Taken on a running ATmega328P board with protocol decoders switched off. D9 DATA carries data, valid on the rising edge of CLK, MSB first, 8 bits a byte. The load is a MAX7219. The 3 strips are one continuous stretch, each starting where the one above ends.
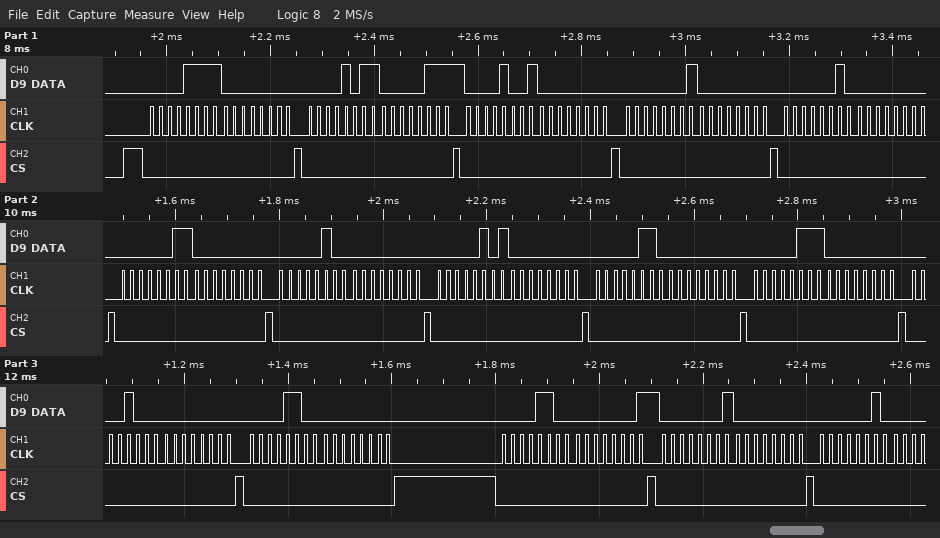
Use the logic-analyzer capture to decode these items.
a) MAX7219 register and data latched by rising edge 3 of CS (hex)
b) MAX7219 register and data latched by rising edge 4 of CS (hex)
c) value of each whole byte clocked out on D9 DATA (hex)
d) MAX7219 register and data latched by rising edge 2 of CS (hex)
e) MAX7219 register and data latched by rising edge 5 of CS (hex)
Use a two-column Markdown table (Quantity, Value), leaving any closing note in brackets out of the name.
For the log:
| Quantity | Value |
|---|---|
| MAX7219 register and data latched by rising edge 3 of CS | register 0xB, data 0x07 |
| MAX7219 register and data latched by rising edge 4 of CS | register 0x9, data 0x00 |
| value of each whole byte clocked out on D9 DATA | 0F 00 0B 07 09 00 01 00 02 00 03 00 04 00 05 00 06 00 07 00 08 00 0C 00 0C 01 01 00 02 |
| MAX7219 register and data latched by rising edge 2 of CS | register 0xF, data 0x00 |
| MAX7219 register and data latched by rising edge 5 of CS | register 0x1, data 0x00 |
